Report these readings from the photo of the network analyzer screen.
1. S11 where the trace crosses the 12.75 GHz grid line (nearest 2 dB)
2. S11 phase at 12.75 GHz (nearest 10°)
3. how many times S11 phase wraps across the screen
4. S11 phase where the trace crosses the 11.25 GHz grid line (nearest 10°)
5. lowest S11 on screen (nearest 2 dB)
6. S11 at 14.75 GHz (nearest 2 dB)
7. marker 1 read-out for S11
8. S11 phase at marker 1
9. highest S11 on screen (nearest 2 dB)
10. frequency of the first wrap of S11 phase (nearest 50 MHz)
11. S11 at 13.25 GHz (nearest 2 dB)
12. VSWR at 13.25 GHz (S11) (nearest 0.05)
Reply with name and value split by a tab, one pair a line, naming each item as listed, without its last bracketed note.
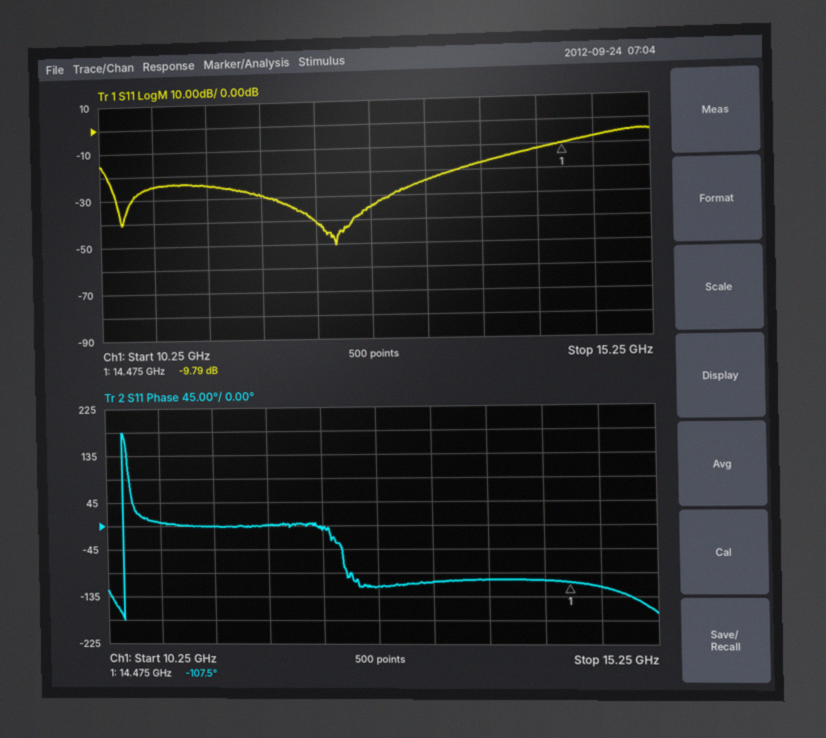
S11 where the trace crosses the 12.75 GHz grid line	-34 dB
S11 phase at 12.75 GHz	-120°
how many times S11 phase wraps across the screen	1
S11 phase where the trace crosses the 11.25 GHz grid line	0°
lowest S11 on screen	-50 dB
S11 at 14.75 GHz	-8 dB
marker 1 read-out for S11	-9.79 dB
S11 phase at marker 1	-107.5°
highest S11 on screen	-4 dB
frequency of the first wrap of S11 phase	10.40 GHz
S11 at 13.25 GHz	-24 dB
VSWR at 13.25 GHz (S11)	1.15
